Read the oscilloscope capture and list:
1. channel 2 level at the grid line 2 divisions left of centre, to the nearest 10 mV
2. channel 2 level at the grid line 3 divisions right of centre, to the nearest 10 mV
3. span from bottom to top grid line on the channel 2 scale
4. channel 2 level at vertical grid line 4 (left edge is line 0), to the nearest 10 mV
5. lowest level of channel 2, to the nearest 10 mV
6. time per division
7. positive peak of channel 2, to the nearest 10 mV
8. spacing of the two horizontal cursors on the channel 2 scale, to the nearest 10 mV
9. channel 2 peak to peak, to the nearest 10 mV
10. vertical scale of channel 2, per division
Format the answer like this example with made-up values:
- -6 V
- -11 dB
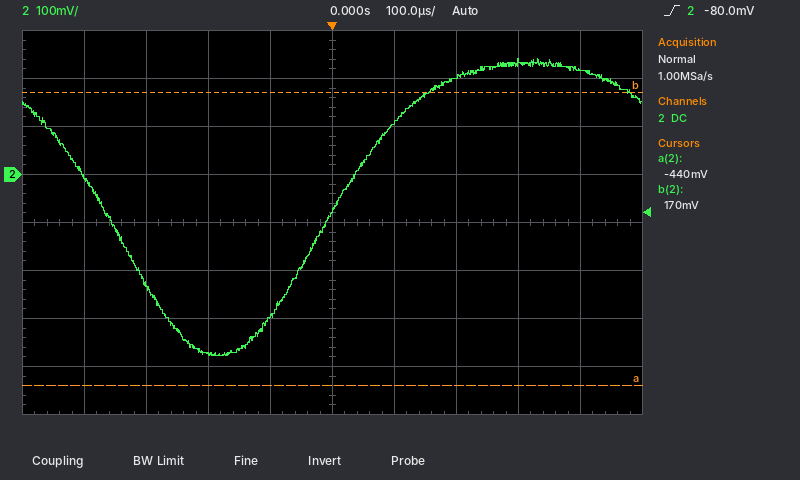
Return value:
- -370 mV
- 230 mV
- 800 mV
- -300 mV
- -380 mV
- 100 µs
- 240 mV
- 610 mV
- 620 mV
- 100 mV
